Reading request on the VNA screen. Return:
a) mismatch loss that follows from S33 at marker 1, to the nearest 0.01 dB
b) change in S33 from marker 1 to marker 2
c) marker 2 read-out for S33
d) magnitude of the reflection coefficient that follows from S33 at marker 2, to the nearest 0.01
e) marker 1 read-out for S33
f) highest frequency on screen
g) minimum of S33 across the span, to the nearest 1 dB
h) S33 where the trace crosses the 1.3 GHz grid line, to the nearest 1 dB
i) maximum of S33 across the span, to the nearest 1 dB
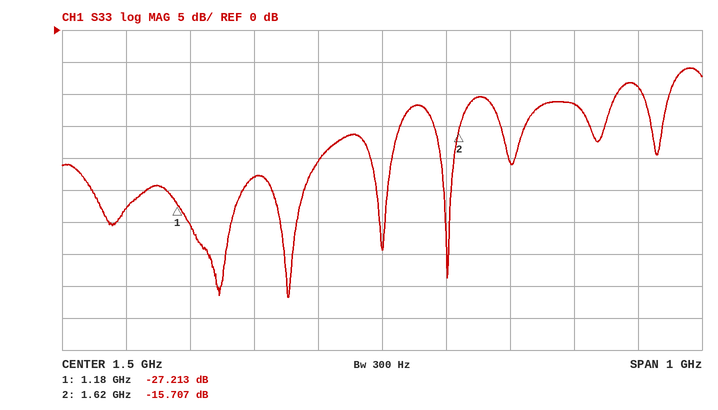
0.01 dB
11.506 dB
-15.707 dB
0.16
-27.213 dB
2 GHz
-42 dB
-23 dB
-6 dB
